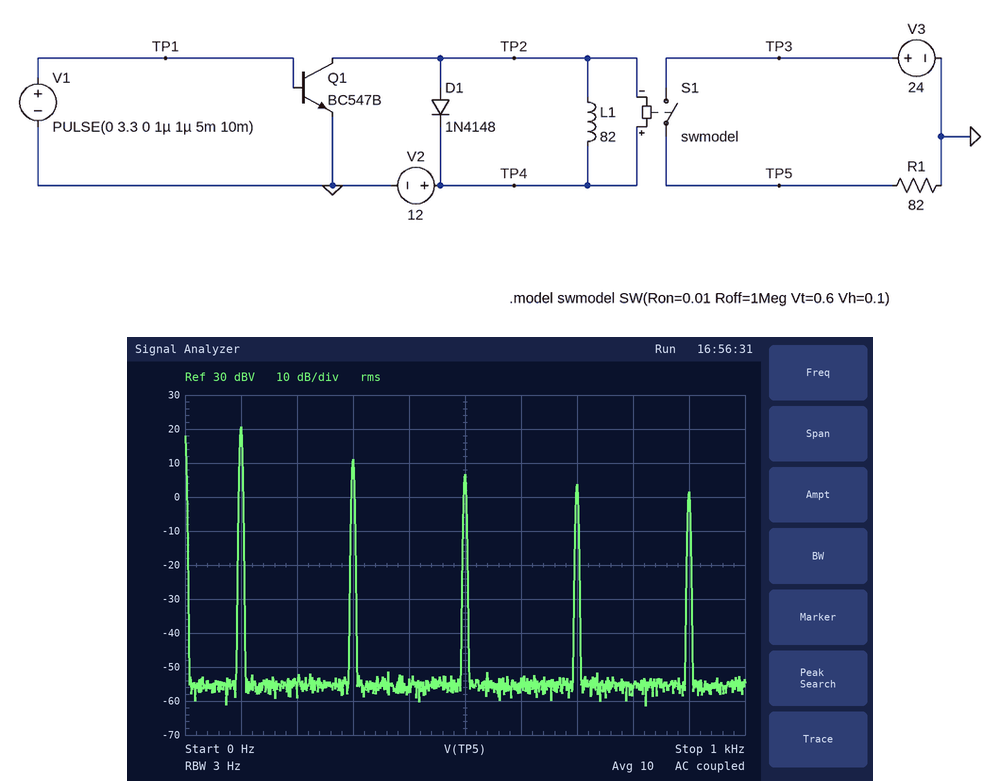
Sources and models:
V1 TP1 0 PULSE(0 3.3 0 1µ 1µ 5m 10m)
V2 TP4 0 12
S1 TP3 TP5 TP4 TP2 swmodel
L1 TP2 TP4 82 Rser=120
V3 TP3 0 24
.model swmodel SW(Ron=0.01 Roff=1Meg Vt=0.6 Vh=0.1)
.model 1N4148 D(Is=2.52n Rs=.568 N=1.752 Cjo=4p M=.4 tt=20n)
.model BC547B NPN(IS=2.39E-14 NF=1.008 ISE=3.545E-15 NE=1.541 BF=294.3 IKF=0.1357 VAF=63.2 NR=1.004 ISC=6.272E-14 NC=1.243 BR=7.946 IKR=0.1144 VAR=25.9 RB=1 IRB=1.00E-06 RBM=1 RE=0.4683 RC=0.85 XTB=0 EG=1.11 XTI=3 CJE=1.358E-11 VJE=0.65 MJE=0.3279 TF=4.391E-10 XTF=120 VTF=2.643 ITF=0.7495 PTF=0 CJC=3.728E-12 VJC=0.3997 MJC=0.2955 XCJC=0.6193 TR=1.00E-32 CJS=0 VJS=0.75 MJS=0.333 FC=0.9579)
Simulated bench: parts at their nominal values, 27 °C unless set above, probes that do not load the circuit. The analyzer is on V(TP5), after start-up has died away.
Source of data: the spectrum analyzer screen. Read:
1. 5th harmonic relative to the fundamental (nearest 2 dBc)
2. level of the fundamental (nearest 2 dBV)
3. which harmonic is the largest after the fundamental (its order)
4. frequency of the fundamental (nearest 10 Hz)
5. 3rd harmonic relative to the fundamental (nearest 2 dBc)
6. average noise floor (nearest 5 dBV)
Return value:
-14 dBc
20 dBV
3
100 Hz
-10 dBc
-55 dBV
